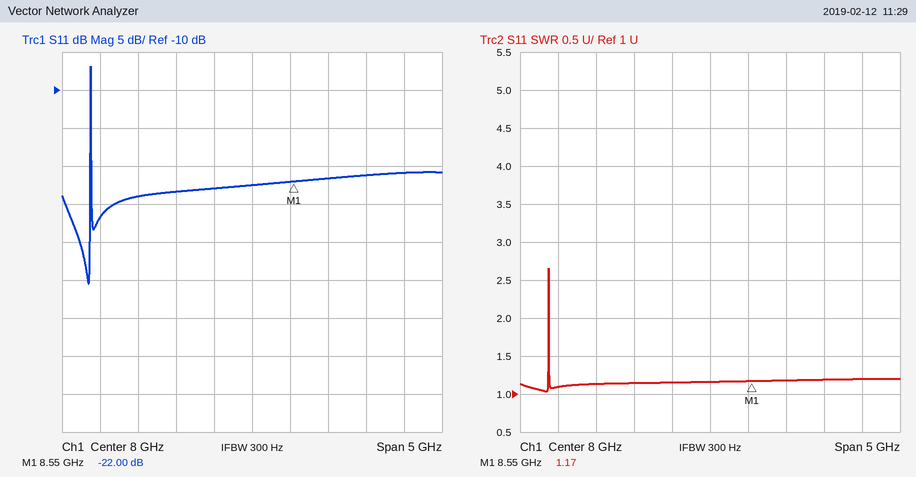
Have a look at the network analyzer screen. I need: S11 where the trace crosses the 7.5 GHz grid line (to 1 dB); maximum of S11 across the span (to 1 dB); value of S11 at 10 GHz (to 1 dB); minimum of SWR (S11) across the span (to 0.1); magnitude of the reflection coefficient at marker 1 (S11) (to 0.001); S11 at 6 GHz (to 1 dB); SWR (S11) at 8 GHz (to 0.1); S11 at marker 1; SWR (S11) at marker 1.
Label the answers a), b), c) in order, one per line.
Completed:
a) -23 dB
b) -7 dB
c) -21 dB
d) 1.0
e) 0.079
f) -27 dB
g) 1.2
h) -22.00 dB
i) 1.17
